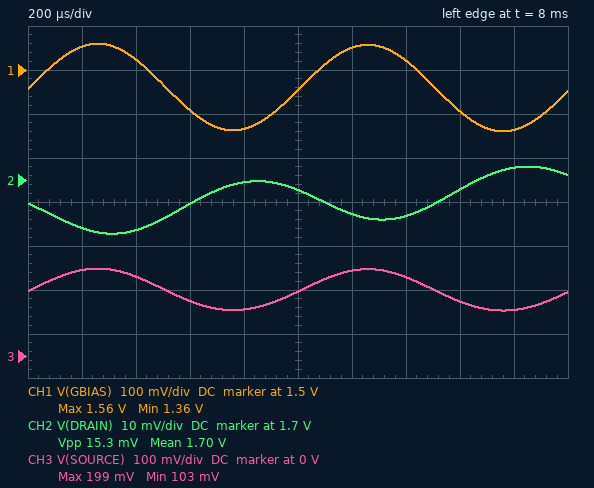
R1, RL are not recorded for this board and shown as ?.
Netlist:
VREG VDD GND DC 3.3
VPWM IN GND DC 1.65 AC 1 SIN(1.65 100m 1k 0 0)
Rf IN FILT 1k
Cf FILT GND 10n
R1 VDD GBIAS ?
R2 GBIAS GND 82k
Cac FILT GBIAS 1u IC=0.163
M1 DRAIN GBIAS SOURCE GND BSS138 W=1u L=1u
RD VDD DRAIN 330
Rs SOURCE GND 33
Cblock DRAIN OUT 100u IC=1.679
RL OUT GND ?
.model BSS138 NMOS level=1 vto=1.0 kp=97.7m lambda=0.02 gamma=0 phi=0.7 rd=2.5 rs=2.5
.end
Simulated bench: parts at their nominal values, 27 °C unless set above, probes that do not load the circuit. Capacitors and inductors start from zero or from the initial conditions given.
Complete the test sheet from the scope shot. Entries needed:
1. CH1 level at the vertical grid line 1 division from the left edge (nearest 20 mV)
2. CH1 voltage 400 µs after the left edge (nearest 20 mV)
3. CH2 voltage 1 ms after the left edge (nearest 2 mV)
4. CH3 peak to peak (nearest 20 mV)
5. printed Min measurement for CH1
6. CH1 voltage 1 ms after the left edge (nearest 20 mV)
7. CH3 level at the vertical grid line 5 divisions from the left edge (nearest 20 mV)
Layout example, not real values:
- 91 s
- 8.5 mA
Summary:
- 1.56 V
- 1.52 V
- 1.698 V
- 100 mV
- 1.36 V
- 1.46 V
- 140 mV
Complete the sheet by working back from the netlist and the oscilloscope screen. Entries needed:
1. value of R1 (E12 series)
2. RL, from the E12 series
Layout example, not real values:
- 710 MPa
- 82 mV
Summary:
- 120 kΩ
- 3.3 Ω
